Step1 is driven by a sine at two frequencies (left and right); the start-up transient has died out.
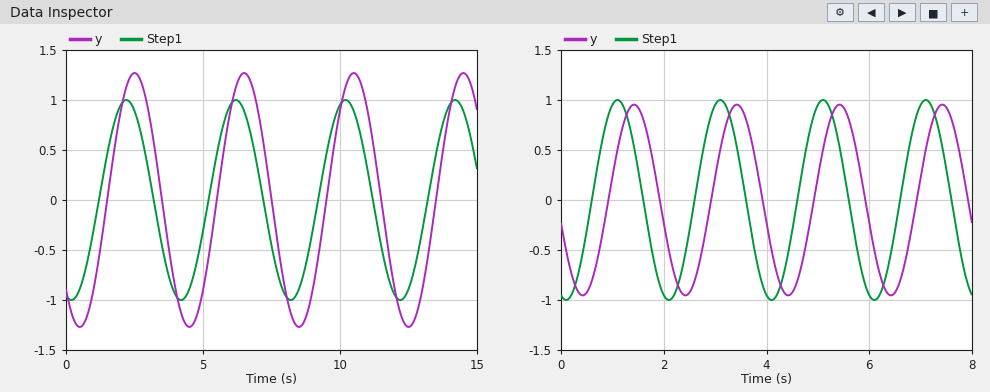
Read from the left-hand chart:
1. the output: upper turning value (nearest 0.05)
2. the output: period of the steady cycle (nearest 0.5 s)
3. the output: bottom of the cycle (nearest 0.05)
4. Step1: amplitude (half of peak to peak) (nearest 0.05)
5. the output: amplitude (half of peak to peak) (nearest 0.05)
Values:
1.25
4.0 s
-1.25
1.00
1.25
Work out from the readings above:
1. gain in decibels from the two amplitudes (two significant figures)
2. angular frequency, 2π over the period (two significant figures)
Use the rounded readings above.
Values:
1.9 dB
1.6 rad/s
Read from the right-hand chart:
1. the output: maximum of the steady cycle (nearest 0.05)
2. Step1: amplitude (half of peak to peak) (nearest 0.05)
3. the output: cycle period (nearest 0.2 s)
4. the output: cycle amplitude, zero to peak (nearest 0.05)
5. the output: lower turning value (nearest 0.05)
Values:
0.95
1.00
2.0 s
0.95
-0.95
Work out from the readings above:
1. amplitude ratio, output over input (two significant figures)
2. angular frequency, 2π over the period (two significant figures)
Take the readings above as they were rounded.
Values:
0.95
3.1 rad/s
